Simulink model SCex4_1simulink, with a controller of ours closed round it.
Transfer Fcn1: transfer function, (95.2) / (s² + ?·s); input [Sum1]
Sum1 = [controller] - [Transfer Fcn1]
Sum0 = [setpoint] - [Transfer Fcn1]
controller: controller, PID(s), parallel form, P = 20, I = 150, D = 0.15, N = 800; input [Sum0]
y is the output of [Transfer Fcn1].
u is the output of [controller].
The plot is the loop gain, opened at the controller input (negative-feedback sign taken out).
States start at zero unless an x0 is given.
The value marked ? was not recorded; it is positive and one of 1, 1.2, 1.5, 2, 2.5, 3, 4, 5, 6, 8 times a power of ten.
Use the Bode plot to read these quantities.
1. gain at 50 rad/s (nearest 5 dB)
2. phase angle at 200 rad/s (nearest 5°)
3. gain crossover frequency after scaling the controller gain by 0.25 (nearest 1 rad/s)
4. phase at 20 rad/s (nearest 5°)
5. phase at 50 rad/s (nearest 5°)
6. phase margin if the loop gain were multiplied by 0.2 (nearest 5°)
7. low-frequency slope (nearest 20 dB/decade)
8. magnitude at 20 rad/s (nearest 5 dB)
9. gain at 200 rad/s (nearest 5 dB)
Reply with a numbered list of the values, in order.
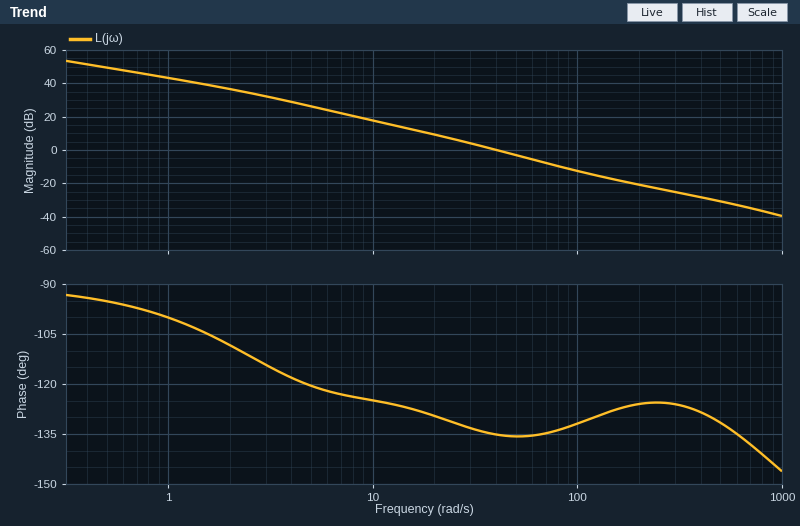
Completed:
1. -5 dB
2. -125°
3. 16 rad/s
4. -130°
5. -135°
6. 55°
7. -20 dB/decade
8. 10 dB
9. -20 dB
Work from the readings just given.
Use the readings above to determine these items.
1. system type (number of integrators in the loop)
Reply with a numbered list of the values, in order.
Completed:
1. 1
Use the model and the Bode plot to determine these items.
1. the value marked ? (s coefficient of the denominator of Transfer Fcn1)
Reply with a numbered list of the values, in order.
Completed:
1. 30
